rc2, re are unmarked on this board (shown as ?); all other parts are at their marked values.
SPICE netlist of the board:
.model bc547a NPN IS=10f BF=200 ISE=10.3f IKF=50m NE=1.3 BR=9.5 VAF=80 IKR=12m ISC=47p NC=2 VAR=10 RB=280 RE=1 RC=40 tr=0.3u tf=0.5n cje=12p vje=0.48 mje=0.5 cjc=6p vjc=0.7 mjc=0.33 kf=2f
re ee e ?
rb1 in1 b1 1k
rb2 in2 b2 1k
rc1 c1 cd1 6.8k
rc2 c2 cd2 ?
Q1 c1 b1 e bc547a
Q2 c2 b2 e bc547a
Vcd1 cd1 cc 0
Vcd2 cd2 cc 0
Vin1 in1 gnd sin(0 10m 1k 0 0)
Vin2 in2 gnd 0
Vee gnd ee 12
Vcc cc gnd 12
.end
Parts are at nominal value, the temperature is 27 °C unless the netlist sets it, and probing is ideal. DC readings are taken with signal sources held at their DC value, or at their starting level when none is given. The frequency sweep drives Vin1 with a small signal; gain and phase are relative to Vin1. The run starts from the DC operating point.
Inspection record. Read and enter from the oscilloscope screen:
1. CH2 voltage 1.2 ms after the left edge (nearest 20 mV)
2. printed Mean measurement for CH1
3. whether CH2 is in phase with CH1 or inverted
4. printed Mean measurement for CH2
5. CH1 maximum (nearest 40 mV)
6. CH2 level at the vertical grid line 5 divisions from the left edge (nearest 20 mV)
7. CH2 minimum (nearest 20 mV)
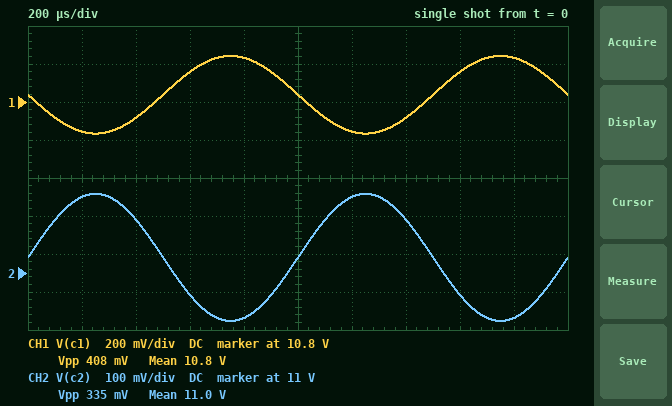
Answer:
11.20 V
10.8 V
inverted
11.0 V
11.04 V
11.04 V
10.88 V
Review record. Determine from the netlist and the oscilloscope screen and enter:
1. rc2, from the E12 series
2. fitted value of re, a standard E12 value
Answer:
5.6 kΩ
33 kΩ
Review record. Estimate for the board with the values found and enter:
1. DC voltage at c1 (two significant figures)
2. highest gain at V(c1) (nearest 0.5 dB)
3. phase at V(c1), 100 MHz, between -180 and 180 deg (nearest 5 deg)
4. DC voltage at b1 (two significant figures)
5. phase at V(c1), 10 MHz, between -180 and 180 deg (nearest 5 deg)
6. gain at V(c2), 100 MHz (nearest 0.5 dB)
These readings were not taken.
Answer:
11 V
26.5 dB
5 deg
-1.5 mV
75 deg
-9.5 dB
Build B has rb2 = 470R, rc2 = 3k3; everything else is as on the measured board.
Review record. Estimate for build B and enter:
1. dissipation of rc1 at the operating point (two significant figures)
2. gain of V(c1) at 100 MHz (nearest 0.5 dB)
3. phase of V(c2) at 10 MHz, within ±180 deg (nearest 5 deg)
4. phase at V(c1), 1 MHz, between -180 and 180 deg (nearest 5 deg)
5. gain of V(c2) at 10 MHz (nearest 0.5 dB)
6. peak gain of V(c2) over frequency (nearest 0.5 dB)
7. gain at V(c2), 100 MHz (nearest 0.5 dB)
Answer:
190 µW
-8.0 dB
-80 deg
140 deg
2.5 dB
20.0 dB
-13.5 dB
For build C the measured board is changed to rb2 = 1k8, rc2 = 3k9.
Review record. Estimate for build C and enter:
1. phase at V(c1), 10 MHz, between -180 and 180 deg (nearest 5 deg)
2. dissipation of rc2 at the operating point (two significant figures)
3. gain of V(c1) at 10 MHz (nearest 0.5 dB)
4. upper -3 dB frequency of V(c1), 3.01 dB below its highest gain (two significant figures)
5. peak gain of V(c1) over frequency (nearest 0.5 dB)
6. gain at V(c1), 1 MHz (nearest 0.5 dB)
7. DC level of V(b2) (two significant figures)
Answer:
70 deg
110 µW
5.5 dB
870 kHz
26.0 dB
22.5 dB
-2.7 mV
